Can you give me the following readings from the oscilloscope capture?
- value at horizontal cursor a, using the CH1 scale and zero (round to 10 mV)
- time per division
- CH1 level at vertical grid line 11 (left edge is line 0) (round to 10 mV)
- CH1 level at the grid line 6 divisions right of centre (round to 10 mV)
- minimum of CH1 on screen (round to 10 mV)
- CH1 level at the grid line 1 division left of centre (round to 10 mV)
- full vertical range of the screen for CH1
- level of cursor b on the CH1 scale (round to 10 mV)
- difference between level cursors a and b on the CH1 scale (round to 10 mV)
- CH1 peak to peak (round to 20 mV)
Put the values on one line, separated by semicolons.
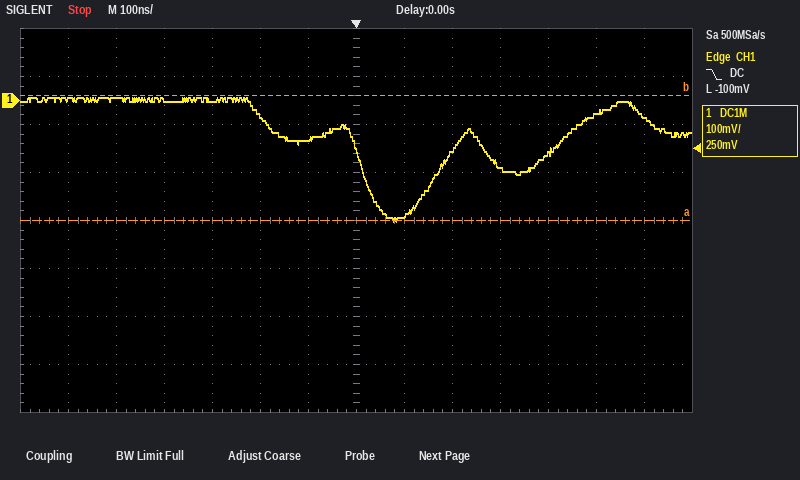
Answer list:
-250 mV; 100 ns; -110 mV; -30 mV; -250 mV; -80 mV; 800 mV; 10 mV; 260 mV; 260 mV
